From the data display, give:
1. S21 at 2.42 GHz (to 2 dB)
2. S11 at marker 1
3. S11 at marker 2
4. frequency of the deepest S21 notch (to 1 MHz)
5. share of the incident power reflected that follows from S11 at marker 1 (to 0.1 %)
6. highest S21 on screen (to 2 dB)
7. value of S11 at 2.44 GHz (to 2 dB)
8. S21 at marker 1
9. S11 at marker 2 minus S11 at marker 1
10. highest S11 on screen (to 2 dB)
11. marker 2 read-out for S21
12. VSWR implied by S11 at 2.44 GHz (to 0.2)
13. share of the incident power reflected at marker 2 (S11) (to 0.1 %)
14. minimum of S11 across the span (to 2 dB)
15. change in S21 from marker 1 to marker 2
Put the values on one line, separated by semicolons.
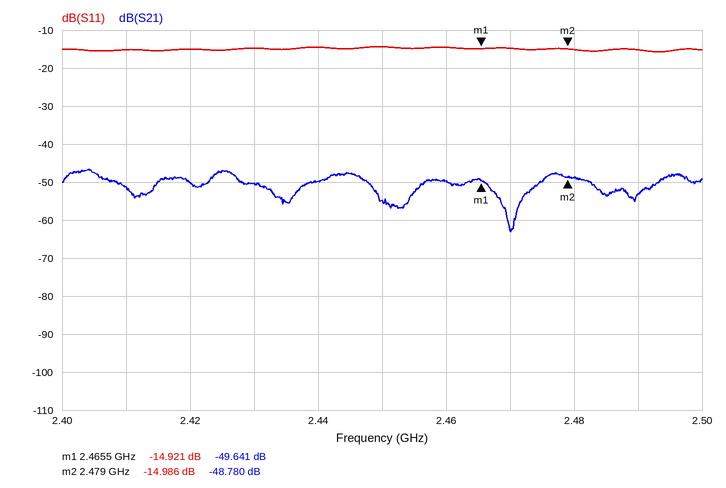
-50 dB; -14.921 dB; -14.986 dB; 2.470 GHz; 3.2 %; -46 dB; -14 dB; -49.641 dB; -0.065 dB; -14 dB; -48.780 dB; 1.4; 3.2 %; -16 dB; 0.861 dB
